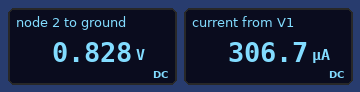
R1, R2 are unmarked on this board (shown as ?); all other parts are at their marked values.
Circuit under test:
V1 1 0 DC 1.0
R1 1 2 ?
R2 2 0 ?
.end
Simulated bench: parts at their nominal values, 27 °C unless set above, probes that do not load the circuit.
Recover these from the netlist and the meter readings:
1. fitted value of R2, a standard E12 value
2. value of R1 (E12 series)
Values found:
2.7 kΩ
560 Ω
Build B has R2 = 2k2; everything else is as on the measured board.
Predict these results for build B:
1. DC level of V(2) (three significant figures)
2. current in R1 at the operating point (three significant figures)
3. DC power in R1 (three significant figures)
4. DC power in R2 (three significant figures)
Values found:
797 mV
362 µA
73.5 µW
289 µW
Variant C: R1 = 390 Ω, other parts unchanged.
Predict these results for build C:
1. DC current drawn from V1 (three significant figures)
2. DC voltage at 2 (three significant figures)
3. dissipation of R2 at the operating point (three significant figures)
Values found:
324 µA
874 mV
283 µW
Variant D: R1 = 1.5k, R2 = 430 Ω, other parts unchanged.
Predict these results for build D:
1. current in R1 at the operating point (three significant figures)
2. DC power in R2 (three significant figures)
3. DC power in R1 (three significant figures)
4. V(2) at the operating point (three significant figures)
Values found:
518 µA
115 µW
403 µW
223 mV
